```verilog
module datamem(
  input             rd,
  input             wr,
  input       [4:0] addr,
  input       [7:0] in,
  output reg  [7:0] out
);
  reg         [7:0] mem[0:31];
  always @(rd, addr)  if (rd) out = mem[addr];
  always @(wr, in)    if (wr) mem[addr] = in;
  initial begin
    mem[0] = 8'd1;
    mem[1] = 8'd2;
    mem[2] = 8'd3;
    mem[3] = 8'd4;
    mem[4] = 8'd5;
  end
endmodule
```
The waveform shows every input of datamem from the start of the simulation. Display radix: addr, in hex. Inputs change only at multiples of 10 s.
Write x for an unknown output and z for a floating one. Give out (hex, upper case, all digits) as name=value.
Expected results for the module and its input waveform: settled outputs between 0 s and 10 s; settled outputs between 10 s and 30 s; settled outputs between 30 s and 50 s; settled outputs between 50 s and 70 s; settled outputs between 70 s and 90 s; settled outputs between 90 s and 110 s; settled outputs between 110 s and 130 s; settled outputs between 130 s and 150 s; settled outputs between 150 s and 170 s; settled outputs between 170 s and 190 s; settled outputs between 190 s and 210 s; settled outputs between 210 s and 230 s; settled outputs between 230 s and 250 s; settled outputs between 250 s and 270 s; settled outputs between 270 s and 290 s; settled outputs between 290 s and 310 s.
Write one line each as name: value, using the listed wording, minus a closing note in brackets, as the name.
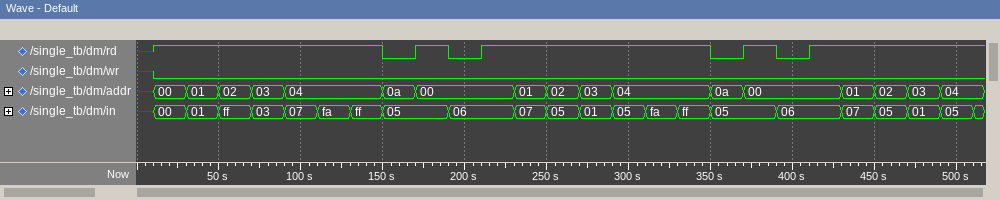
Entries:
settled outputs between 0 s and 10 s: out=x
settled outputs between 10 s and 30 s: out=01
settled outputs between 30 s and 50 s: out=02
settled outputs between 50 s and 70 s: out=03
settled outputs between 70 s and 90 s: out=04
settled outputs between 90 s and 110 s: out=05
settled outputs between 110 s and 130 s: out=05
settled outputs between 130 s and 150 s: out=05
settled outputs between 150 s and 170 s: out=05
settled outputs between 170 s and 190 s: out=01
settled outputs between 190 s and 210 s: out=01
settled outputs between 210 s and 230 s: out=01
settled outputs between 230 s and 250 s: out=02
settled outputs between 250 s and 270 s: out=03
settled outputs between 270 s and 290 s: out=04
settled outputs between 290 s and 310 s: out=05
